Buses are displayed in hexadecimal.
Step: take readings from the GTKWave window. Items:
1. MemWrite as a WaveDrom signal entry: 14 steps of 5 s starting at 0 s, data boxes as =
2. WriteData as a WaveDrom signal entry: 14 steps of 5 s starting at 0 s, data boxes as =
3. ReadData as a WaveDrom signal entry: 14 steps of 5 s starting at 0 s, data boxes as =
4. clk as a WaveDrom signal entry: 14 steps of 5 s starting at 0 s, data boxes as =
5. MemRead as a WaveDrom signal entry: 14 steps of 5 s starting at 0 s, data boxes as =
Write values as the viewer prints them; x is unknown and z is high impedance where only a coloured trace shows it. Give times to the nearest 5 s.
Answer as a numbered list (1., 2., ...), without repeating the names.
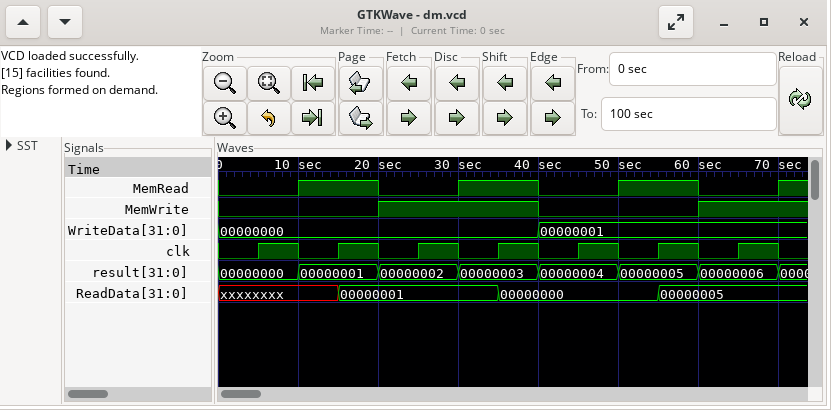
1. {name: 'MemWrite', wave: '0...1...0...1.'}
2. {name: 'WriteData', wave: '=.......=.....', data: '00000000 00000001'}
3. {name: 'ReadData', wave: 'x..=...=...=..', data: '00000001 00000000 00000005'}
4. {name: 'clk', wave: '01010101010101'}
5. {name: 'MemRead', wave: '0.1.0.1.0.1.0.'}
